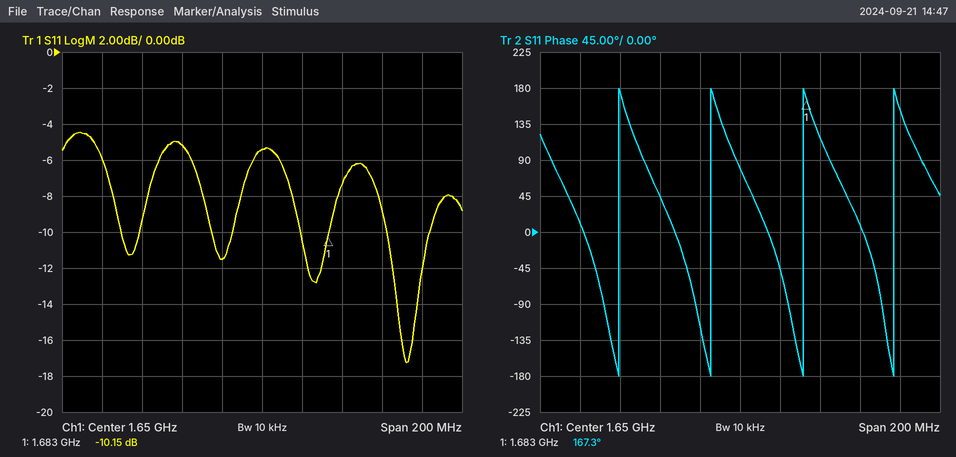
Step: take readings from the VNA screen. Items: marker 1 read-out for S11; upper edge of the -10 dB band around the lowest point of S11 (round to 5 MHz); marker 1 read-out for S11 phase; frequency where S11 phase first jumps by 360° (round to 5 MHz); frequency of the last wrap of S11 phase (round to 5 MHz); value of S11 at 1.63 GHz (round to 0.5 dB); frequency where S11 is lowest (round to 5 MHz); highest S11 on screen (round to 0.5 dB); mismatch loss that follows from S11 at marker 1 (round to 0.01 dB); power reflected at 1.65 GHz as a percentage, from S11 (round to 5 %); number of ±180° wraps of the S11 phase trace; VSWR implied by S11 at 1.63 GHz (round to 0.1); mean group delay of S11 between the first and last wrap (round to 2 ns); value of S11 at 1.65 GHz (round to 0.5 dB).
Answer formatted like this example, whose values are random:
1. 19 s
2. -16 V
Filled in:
1. -10.15 dB
2. 1.735 GHz
3. 167.3°
4. 1.590 GHz
5. 1.725 GHz
6. -11.5 dB
7. 1.720 GHz
8. -4.5 dB
9. 0.44 dB
10. 30 %
11. 4
12. 1.7
13. 22 ns
14. -5.5 dB
